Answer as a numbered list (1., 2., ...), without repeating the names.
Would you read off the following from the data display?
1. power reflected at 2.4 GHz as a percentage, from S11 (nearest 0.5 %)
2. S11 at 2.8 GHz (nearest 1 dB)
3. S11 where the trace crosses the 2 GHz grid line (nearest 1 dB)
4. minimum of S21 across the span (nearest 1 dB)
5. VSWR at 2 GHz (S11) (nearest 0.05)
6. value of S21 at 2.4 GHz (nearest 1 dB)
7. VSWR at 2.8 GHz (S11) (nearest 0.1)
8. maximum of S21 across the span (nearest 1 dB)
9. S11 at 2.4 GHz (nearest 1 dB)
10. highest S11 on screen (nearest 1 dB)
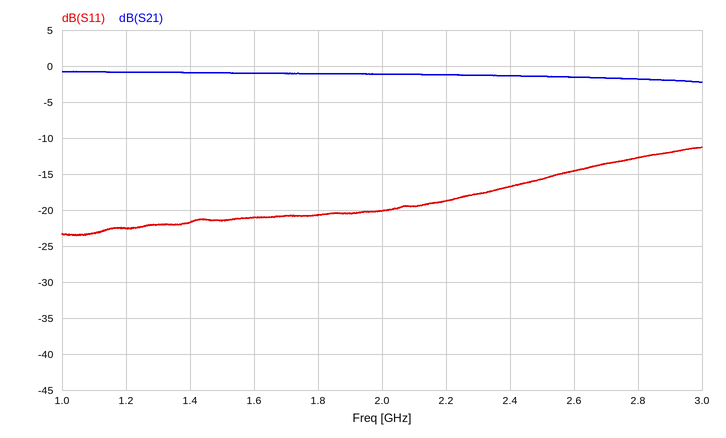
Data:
1. 2.0 %
2. -13 dB
3. -20 dB
4. -2 dB
5. 1.20
6. -1 dB
7. 1.6
8. -1 dB
9. -17 dB
10. -11 dB
